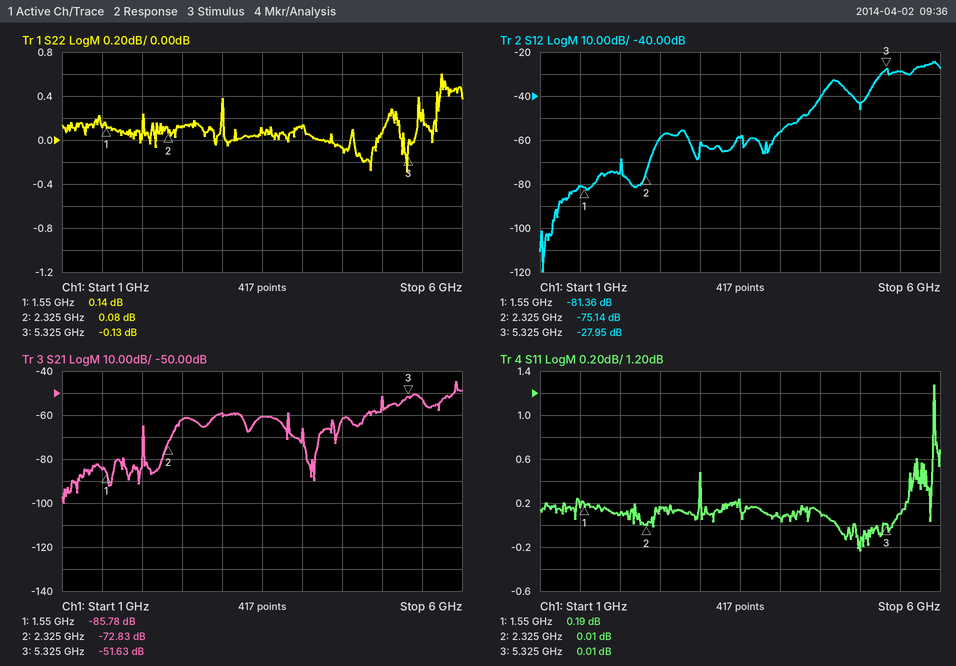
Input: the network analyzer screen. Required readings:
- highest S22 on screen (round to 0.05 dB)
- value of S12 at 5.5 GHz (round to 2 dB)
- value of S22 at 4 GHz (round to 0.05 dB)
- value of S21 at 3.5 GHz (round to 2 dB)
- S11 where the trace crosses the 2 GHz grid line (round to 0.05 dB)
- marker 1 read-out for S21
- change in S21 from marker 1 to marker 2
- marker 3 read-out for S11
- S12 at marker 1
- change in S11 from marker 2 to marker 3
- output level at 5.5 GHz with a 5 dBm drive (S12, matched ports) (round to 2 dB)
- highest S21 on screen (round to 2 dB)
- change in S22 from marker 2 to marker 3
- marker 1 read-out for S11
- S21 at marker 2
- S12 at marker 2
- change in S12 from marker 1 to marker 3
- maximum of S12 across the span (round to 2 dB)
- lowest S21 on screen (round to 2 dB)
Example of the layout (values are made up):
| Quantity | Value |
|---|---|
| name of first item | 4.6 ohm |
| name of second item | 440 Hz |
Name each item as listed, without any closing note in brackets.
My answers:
| Quantity | Value |
|---|---|
| highest S22 on screen | 0.60 dB |
| value of S12 at 5.5 GHz | -28 dB |
| value of S22 at 4 GHz | 0.10 dB |
| value of S21 at 3.5 GHz | -60 dB |
| S11 where the trace crosses the 2 GHz grid line | 0.10 dB |
| marker 1 read-out for S21 | -85.78 dB |
| change in S21 from marker 1 to marker 2 | 12.95 dB |
| marker 3 read-out for S11 | 0.01 dB |
| S12 at marker 1 | -81.36 dB |
| change in S11 from marker 2 to marker 3 | 0.00 dB |
| output level at 5.5 GHz with a 5 dBm drive (S12, matched ports) | -24 dBm |
| highest S21 on screen | -44 dB |
| change in S22 from marker 2 to marker 3 | -0.21 dB |
| marker 1 read-out for S11 | 0.19 dB |
| S21 at marker 2 | -72.83 dB |
| S12 at marker 2 | -75.14 dB |
| change in S12 from marker 1 to marker 3 | 53.41 dB |
| maximum of S12 across the span | -24 dB |
| lowest S21 on screen | -100 dB |
